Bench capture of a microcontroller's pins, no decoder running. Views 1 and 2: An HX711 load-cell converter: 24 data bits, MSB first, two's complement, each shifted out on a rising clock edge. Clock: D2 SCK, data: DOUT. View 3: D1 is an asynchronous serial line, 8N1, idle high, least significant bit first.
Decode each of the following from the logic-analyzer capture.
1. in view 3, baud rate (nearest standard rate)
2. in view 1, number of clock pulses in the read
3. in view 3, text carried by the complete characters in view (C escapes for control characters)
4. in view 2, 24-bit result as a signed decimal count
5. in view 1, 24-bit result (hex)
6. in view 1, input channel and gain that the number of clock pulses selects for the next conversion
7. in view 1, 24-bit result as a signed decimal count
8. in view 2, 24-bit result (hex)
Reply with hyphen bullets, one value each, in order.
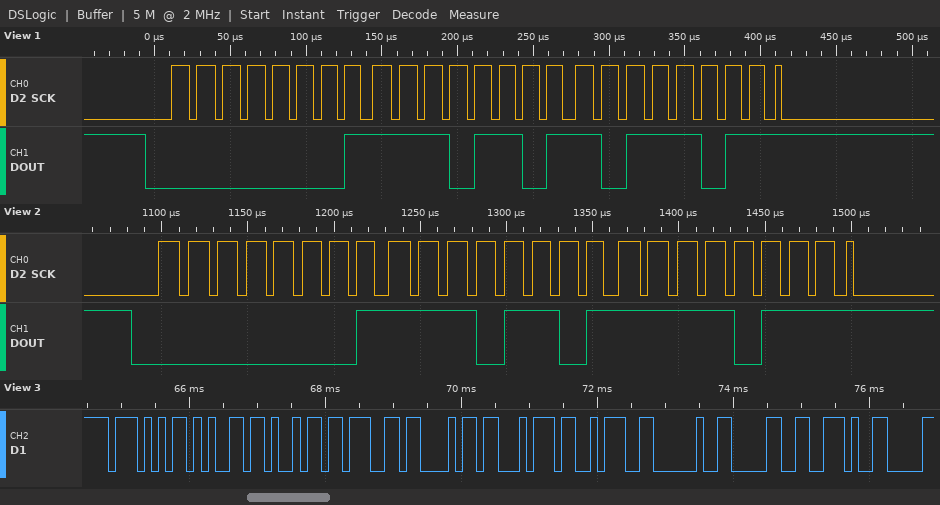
- 9600 baud
- 25
- "Weight: 0."
- 126455
- 0x01EDBB
- channel A, gain 128
- 126395
- 0x01EDF7
